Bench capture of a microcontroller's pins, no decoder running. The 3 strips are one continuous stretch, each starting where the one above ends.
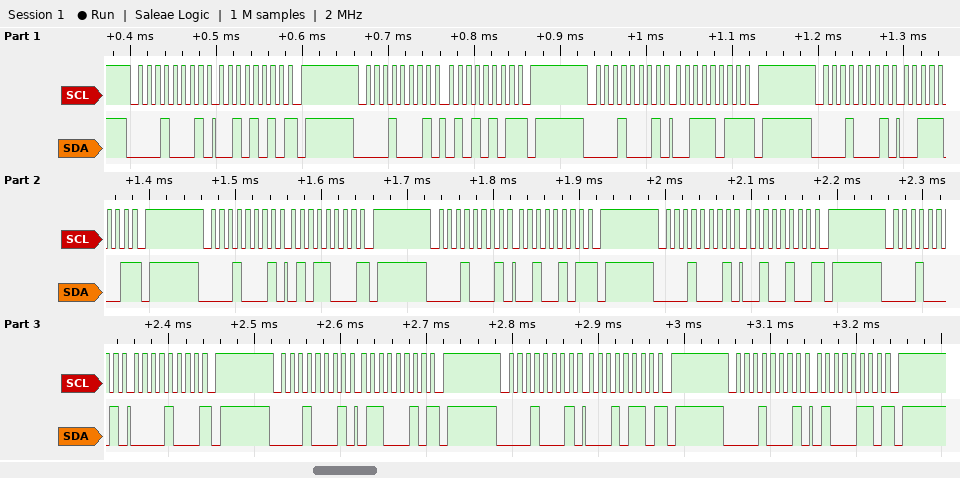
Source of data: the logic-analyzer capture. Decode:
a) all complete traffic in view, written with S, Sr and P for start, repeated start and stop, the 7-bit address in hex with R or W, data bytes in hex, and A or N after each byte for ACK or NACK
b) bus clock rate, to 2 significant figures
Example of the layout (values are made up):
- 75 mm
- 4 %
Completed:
- S 08R A 2A N P S 08R A 55 N P S 08R A 3B N P S 08R A 39 N P S 08R A 58 N P S 08R A 25 N P S 08R A 24 N P S 08R A 08 N P S 08R A 62 N P S 08R A 16 N P S 08R A 46 N P
- 100 kHz
